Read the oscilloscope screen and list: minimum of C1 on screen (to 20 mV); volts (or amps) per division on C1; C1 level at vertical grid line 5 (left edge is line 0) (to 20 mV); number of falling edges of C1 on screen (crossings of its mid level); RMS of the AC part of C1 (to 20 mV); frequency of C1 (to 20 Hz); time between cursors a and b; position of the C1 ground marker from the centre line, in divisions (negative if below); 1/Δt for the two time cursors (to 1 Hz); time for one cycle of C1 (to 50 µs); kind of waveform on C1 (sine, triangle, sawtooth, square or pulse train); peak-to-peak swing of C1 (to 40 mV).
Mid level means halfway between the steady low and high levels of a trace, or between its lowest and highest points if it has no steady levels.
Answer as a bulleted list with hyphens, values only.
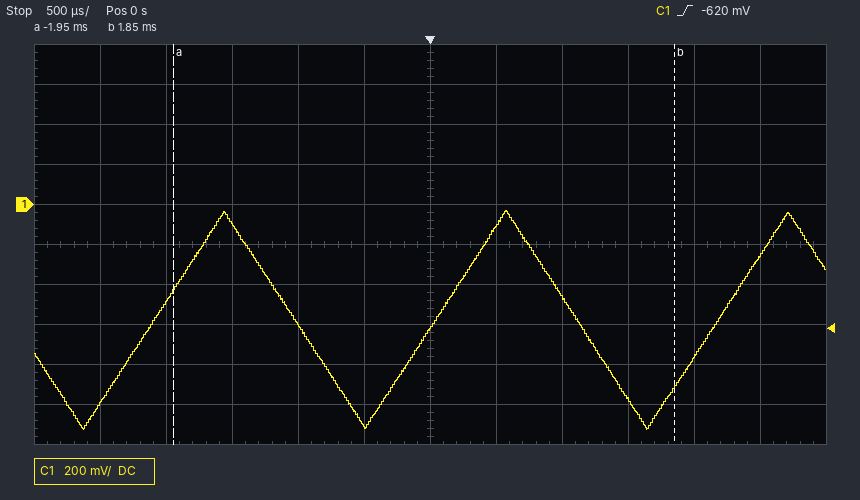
- -1.12 V
- 200 mV
- -1.10 V
- 2
- 320 mV
- 460 Hz
- 3.80 ms
- +1.0 div
- 263 Hz
- 2.15 ms
- triangle
- 1.08 V
